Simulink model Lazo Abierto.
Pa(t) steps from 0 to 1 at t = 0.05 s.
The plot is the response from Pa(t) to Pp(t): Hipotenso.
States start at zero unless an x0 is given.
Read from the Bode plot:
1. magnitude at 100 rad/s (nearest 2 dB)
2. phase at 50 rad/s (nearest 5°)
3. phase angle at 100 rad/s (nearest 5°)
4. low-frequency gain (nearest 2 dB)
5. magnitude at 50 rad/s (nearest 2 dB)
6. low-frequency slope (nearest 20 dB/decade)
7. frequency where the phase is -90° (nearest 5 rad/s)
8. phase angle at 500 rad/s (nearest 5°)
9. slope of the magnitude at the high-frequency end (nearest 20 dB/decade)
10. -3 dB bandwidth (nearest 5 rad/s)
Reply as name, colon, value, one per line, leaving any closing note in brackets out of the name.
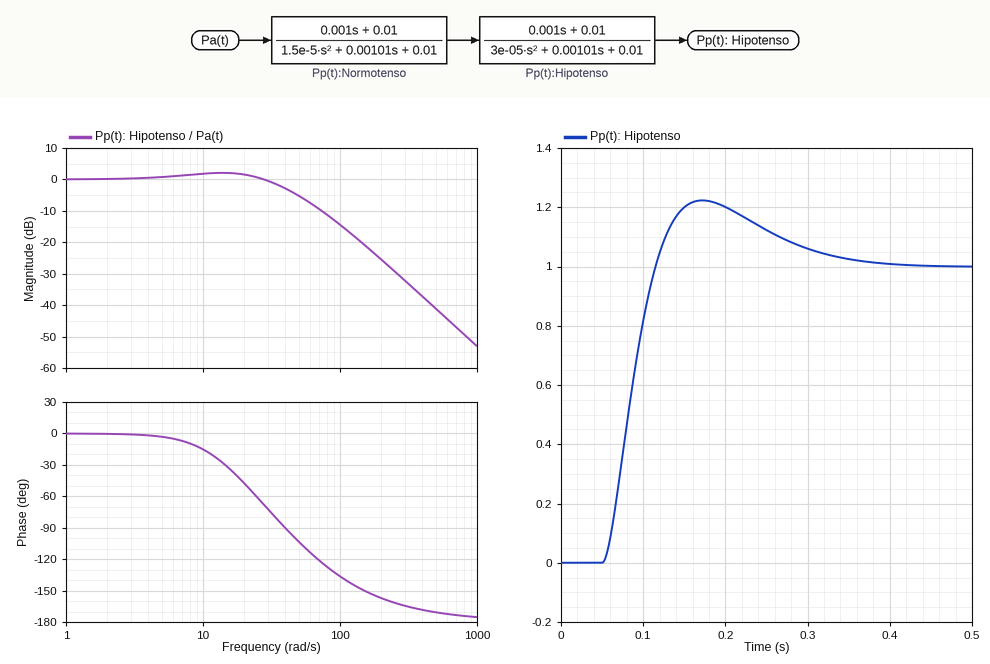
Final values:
magnitude at 100 rad/s: -14 dB
phase at 50 rad/s: -105°
phase angle at 100 rad/s: -135°
low-frequency gain: 0 dB
magnitude at 50 rad/s: -6 dB
low-frequency slope: 0 dB/decade
frequency where the phase is -90°: 40 rad/s
phase angle at 500 rad/s: -170°
slope of the magnitude at the high-frequency end: -40 dB/decade
-3 dB bandwidth: 40 rad/s
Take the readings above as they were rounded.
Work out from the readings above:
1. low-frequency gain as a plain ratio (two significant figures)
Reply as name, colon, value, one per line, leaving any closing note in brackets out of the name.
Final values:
low-frequency gain as a plain ratio: 1.0
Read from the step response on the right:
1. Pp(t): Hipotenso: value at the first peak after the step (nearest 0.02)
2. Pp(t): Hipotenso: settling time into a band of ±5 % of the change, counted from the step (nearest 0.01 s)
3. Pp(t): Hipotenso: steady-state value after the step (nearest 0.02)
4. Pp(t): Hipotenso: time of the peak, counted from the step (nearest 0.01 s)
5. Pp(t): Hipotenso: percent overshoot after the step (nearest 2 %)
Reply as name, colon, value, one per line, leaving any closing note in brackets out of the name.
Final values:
Pp(t): Hipotenso: value at the first peak after the step: 1.22
Pp(t): Hipotenso: settling time into a band of ±5 % of the change, counted from the step: 0.26 s
Pp(t): Hipotenso: steady-state value after the step: 1.00
Pp(t): Hipotenso: time of the peak, counted from the step: 0.12 s
Pp(t): Hipotenso: percent overshoot after the step: 22 %
